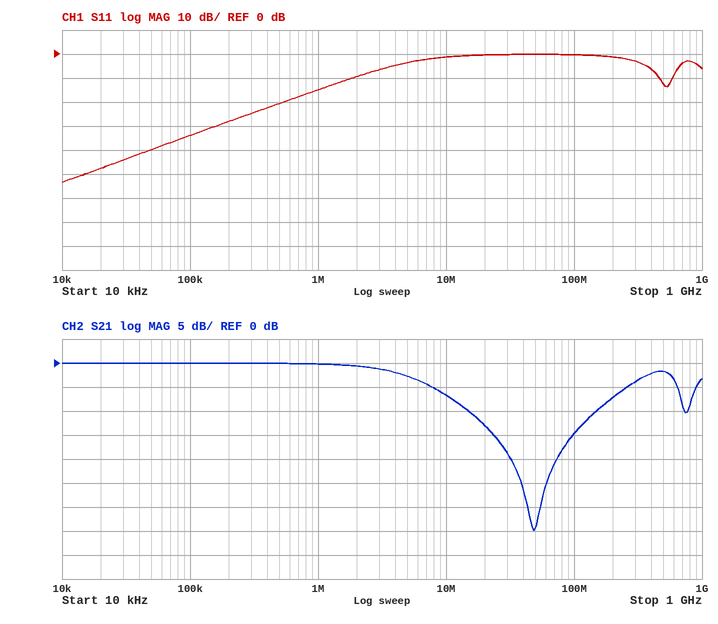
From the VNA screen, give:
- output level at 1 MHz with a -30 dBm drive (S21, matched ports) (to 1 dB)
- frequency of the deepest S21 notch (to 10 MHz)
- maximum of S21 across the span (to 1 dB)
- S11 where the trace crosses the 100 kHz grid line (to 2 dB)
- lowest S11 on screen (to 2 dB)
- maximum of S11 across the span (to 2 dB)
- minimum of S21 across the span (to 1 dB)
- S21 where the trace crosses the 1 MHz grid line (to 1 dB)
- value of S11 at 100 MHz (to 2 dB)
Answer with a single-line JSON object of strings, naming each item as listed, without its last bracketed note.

{"output level at 1 MHz with a -30 dBm drive (S21, matched ports)": "-30 dBm", "frequency of the deepest S21 notch": "50 MHz", "maximum of S21 across the span": "0 dB", "S11 where the trace crosses the 100 kHz grid line": "-34 dB", "lowest S11 on screen": "-54 dB", "maximum of S11 across the span": "0 dB", "minimum of S21 across the span": "-35 dB", "S21 where the trace crosses the 1 MHz grid line": "0 dB", "value of S11 at 100 MHz": "0 dB"}
